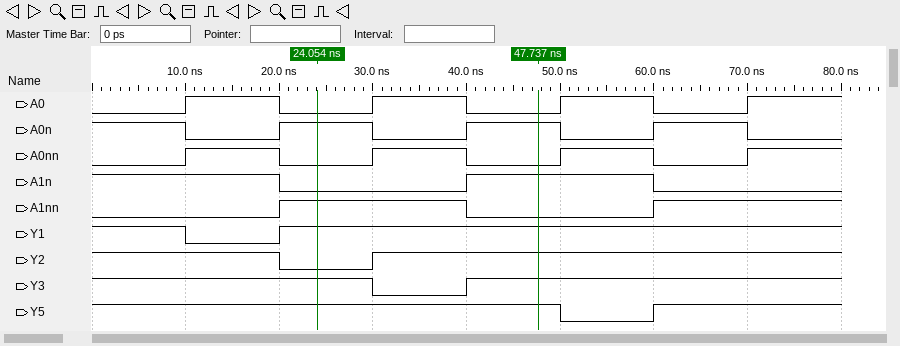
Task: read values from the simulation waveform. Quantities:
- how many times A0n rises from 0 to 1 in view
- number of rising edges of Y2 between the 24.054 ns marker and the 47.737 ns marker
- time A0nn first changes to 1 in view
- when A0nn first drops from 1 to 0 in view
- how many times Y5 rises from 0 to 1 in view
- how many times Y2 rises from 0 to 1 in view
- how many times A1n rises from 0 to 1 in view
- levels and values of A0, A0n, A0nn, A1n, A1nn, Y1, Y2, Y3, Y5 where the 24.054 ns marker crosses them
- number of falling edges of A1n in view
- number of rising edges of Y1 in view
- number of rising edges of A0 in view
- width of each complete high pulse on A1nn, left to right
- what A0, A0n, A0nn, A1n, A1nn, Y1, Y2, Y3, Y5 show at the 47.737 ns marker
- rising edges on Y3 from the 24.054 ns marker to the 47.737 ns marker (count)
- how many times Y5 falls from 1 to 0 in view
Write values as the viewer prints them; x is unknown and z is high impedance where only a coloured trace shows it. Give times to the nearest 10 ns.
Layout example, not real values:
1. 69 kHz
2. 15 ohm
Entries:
1. 3
2. 1
3. 10 ns
4. 20 ns
5. 1
6. 1
7. 1
8. A0=0, A0n=1, A0nn=0, A1n=0, A1nn=1, Y1=1, Y2=0, Y3=1, Y5=1
9. 2
10. 1
11. 4
12. 20 ns
13. A0=0, A0n=1, A0nn=0, A1n=1, A1nn=0, Y1=1, Y2=1, Y3=1, Y5=1
14. 1
15. 1
